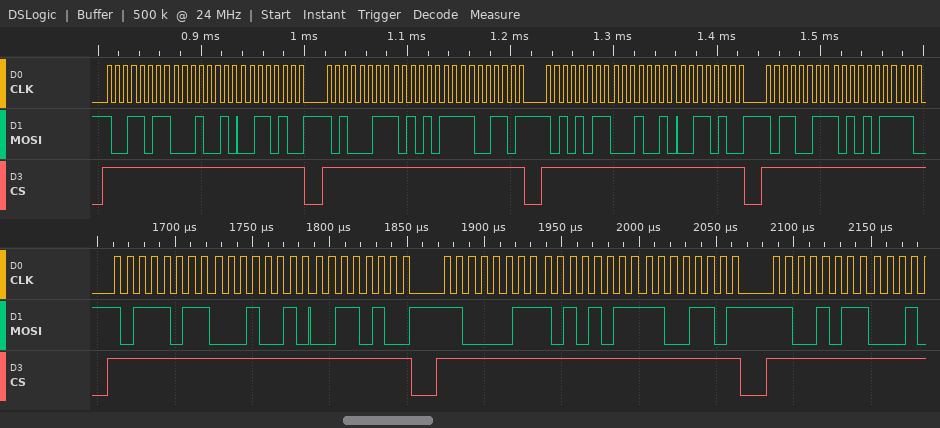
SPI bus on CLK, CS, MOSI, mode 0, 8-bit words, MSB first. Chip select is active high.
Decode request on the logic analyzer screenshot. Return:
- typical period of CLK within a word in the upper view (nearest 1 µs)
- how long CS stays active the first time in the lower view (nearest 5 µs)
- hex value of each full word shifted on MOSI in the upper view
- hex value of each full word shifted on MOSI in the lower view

8 µs
195 µs
9B, 12, 34, A3, AB, CD, AB, 12, 34, B3, AB
BB, 12, 34, C3, AB, CD, CB
